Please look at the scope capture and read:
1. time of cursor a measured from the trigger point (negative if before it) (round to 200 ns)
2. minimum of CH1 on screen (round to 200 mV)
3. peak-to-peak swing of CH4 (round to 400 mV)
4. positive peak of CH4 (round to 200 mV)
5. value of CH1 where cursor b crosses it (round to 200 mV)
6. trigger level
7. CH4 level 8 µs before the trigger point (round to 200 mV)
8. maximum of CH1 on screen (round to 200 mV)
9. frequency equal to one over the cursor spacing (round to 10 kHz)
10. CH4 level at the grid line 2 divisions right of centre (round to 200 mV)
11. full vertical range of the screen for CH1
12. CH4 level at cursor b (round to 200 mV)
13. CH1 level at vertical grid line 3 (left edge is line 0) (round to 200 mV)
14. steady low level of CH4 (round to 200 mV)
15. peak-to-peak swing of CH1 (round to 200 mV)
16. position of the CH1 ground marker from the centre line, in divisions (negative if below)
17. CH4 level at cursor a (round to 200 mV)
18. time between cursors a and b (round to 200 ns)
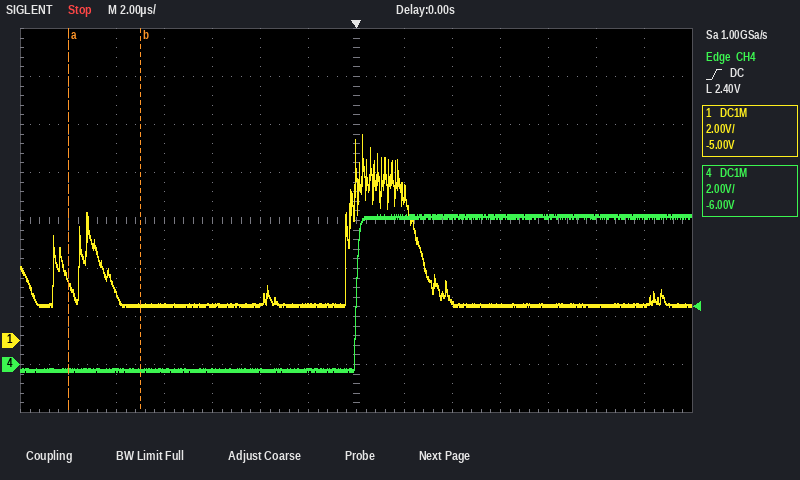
-12.0 µs
1.4 V
6.4 V
6.2 V
1.4 V
2.40 V
-200 mV
8.6 V
330 kHz
6.2 V
16 V
-200 mV
1.4 V
-200 mV
7.2 V
-2.5 div
-200 mV
3.0 µs
